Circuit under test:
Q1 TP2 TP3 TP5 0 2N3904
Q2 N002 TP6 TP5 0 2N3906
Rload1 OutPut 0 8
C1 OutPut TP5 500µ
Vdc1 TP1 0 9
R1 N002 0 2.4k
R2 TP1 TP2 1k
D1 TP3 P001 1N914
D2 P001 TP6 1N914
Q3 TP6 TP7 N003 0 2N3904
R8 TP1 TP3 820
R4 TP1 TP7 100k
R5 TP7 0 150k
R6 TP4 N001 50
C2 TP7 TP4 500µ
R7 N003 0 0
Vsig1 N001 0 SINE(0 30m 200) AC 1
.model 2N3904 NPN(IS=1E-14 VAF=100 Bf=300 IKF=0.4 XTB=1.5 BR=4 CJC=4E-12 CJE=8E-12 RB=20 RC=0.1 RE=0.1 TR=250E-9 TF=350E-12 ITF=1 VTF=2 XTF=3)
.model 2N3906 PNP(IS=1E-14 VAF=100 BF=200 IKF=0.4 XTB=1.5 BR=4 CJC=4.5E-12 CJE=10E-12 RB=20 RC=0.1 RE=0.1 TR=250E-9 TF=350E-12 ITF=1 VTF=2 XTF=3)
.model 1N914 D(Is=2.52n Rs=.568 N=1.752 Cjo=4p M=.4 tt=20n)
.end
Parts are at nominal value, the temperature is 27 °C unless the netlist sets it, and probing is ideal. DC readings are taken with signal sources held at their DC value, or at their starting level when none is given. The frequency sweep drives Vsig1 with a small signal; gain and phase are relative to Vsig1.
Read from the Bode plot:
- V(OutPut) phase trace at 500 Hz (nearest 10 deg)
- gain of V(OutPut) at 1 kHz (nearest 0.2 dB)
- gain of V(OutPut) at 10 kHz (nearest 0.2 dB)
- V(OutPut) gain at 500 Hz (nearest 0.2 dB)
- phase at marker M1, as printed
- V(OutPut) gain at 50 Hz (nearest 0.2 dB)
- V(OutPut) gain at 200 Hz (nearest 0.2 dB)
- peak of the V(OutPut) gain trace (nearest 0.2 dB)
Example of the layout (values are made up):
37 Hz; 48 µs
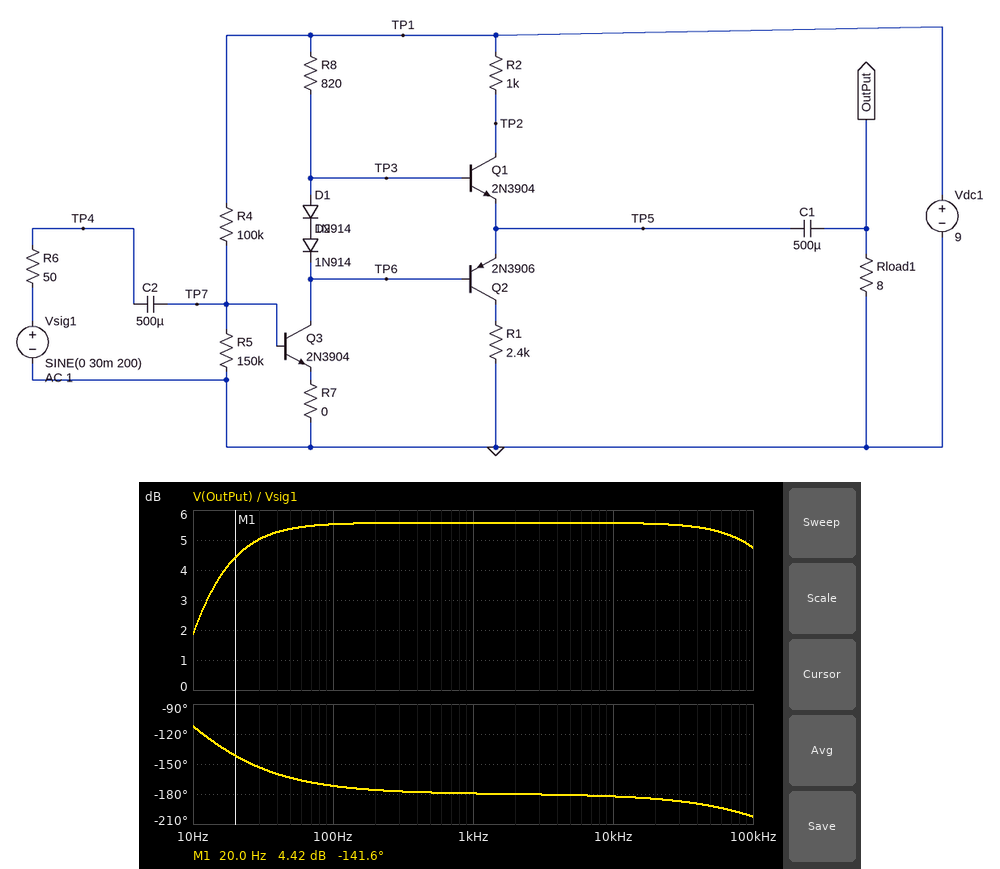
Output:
-180 deg; 5.6 dB; 5.6 dB; 5.6 dB; -141.6 deg; 5.4 dB; 5.6 dB; 5.6 dB
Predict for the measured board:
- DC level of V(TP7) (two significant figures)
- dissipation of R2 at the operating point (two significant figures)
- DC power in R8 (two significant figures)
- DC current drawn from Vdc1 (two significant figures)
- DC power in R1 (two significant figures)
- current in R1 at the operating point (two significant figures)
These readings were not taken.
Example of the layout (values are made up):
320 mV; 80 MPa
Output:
720 mV; 1.8 mW; 69 mW; 11 mA; 280 µW; 340 µA
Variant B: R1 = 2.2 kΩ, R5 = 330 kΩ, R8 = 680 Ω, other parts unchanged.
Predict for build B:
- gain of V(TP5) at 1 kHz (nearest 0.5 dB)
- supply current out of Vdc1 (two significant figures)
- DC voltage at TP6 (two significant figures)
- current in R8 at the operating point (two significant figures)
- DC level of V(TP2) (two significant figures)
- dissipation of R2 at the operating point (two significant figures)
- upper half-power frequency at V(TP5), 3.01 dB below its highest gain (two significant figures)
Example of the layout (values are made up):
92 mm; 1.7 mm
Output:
8.0 dB; 13 mA; 120 mV; 11 mA; 7.3 V; 2.8 mW; 21 Hz
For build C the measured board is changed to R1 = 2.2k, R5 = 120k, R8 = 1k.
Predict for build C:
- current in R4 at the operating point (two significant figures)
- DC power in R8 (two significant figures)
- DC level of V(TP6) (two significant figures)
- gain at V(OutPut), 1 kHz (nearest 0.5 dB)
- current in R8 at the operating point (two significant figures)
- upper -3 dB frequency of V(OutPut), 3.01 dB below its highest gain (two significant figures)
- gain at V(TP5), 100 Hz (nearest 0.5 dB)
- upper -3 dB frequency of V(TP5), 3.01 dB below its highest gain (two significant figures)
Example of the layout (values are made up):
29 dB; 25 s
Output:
83 µA; 57 mW; 100 mV; 3.0 dB; 7.5 mA; 240 kHz; 4.0 dB; 17 Hz
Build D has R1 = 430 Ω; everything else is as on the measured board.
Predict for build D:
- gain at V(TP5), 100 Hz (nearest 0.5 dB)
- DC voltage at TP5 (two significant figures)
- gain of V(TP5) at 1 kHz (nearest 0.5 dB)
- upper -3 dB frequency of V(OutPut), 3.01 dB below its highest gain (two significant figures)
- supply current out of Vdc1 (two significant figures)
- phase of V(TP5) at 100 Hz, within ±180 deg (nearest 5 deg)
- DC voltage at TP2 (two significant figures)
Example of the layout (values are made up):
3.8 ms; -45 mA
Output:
8.0 dB; 810 mV; 7.5 dB; 210 kHz; 12 mA; 170 deg; 6.7 V
